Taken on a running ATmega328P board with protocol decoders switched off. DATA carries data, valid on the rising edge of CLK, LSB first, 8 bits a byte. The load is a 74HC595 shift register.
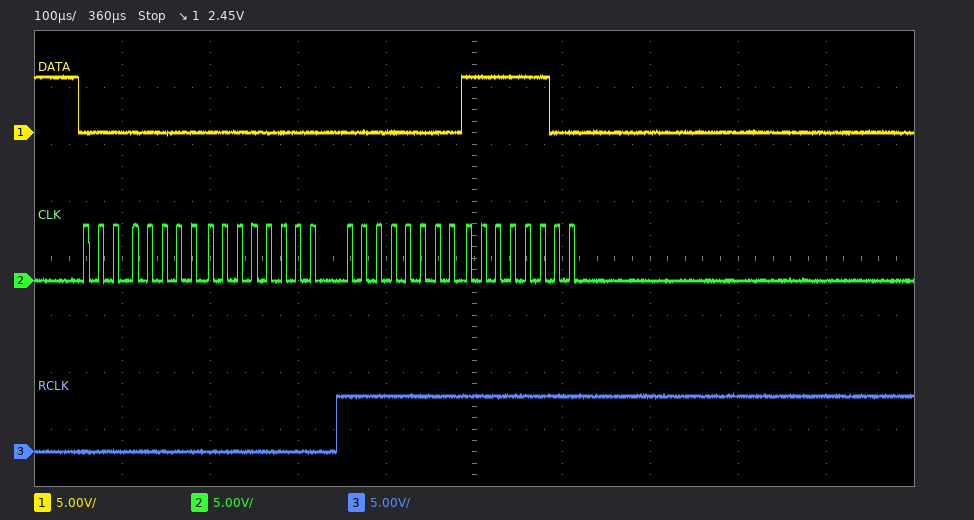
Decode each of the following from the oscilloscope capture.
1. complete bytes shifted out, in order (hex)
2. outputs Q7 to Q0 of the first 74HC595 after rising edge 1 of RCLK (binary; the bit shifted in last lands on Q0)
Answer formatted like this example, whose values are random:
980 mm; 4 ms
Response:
00 00 00 3F; 00000000
